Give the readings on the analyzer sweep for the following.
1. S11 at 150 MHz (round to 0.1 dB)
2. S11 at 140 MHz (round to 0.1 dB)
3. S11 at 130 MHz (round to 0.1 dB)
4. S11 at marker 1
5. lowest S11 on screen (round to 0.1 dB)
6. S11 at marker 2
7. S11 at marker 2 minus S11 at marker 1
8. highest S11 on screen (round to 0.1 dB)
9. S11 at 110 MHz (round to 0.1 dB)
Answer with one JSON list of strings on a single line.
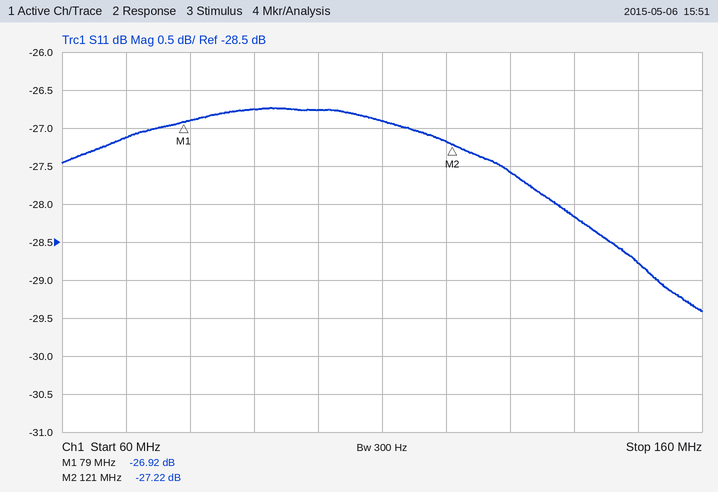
["-28.8 dB", "-28.2 dB", "-27.6 dB", "-26.92 dB", "-29.4 dB", "-27.22 dB", "-0.30 dB", "-26.7 dB", "-26.9 dB"]
